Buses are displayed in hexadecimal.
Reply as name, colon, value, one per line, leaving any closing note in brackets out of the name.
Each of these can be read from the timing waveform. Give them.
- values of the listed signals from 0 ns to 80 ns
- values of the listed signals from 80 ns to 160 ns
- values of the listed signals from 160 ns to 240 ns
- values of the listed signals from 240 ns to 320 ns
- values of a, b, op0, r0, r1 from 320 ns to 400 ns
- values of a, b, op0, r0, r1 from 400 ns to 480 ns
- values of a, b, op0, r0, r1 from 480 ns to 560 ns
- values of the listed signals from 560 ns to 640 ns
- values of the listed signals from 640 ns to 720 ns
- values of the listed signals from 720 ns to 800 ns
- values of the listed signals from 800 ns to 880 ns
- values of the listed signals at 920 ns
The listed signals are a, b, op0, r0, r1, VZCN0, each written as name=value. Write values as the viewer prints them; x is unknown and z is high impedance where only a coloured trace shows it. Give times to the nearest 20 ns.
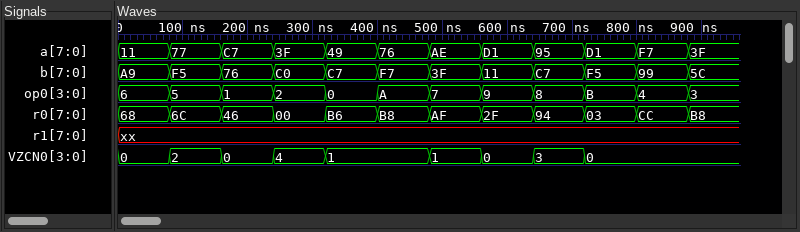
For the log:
values of the listed signals from 0 ns to 80 ns: a=11, b=A9, op0=6, r0=68, r1=xx, VZCN0=0
values of the listed signals from 80 ns to 160 ns: a=77, b=F5, op0=5, r0=6C, r1=xx, VZCN0=2
values of the listed signals from 160 ns to 240 ns: a=C7, b=76, op0=1, r0=46, r1=xx, VZCN0=0
values of the listed signals from 240 ns to 320 ns: a=3F, b=C0, op0=2, r0=00, r1=xx, VZCN0=4
values of a, b, op0, r0, r1 from 320 ns to 400 ns: a=49, b=C7, op0=0, r0=B6, r1=xx
values of a, b, op0, r0, r1 from 400 ns to 480 ns: a=76, b=F7, op0=A, r0=B8, r1=xx
values of a, b, op0, r0, r1 from 480 ns to 560 ns: a=AE, b=3F, op0=7, r0=AF, r1=xx
values of the listed signals from 560 ns to 640 ns: a=D1, b=11, op0=9, r0=2F, r1=xx, VZCN0=0
values of the listed signals from 640 ns to 720 ns: a=95, b=C7, op0=8, r0=94, r1=xx, VZCN0=3
values of the listed signals from 720 ns to 800 ns: a=D1, b=F5, op0=B, r0=03, r1=xx, VZCN0=0
values of the listed signals from 800 ns to 880 ns: a=F7, b=99, op0=4, r0=CC, r1=xx, VZCN0=0
values of the listed signals at 920 ns: a=3F, b=5C, op0=3, r0=B8, r1=xx, VZCN0=0
